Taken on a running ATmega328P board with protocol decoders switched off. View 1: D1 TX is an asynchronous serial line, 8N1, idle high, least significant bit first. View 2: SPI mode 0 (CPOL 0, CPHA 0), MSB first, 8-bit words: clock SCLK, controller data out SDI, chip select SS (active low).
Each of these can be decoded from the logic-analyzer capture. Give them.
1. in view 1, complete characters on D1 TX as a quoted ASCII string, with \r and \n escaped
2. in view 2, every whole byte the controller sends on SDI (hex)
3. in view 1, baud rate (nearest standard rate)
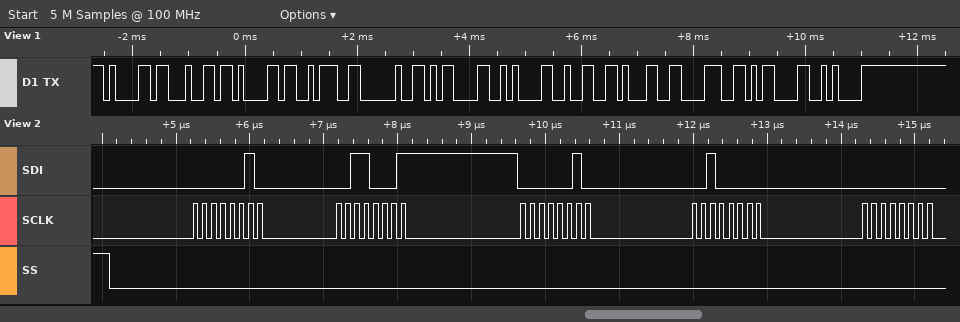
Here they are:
"ada: \r\n218\r\n"
02 31 02 20 00
9600 baud
